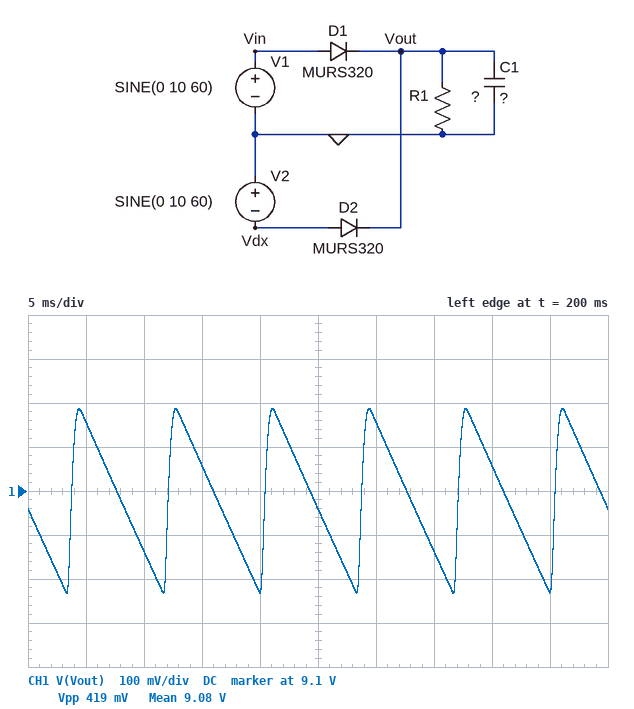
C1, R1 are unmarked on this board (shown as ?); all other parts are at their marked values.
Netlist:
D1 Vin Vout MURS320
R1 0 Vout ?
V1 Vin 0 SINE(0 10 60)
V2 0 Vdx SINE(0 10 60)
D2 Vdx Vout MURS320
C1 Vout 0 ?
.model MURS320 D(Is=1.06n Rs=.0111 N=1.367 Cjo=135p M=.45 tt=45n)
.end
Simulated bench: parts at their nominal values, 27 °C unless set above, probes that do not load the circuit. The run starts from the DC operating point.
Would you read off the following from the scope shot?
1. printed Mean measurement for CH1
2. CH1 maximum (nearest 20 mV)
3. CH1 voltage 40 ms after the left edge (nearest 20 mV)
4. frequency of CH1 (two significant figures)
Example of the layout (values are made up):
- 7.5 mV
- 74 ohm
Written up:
- 9.08 V
- 9.28 V
- 9.16 V
- 120 Hz
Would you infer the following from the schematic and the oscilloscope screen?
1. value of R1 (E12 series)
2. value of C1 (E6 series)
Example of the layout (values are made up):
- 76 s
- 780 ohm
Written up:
- 47 Ω
- 3.3 mF
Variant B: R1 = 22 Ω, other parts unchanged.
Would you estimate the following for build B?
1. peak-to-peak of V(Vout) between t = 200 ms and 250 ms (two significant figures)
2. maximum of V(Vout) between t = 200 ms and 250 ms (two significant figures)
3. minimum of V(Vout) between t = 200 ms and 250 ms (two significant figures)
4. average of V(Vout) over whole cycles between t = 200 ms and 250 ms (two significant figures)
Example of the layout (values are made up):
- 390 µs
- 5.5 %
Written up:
- 840 mV
- 9.3 V
- 8.4 V
- 8.9 V
